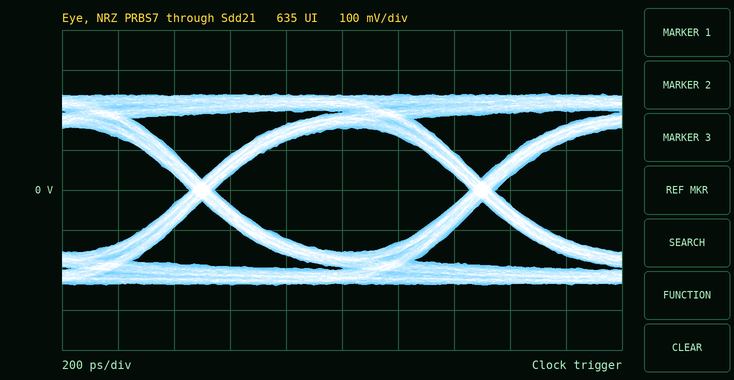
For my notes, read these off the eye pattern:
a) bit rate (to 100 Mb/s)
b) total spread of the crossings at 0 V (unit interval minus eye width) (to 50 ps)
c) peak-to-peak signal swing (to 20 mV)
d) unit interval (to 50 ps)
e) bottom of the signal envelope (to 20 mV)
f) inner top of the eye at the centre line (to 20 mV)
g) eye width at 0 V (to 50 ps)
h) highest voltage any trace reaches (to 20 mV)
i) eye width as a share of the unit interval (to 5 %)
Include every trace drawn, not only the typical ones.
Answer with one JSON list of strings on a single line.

["1.0 Gb/s", "100 ps", "480 mV", "1.00 ns", "-240 mV", "160 mV", "900 ps", "240 mV", "90 %"]
